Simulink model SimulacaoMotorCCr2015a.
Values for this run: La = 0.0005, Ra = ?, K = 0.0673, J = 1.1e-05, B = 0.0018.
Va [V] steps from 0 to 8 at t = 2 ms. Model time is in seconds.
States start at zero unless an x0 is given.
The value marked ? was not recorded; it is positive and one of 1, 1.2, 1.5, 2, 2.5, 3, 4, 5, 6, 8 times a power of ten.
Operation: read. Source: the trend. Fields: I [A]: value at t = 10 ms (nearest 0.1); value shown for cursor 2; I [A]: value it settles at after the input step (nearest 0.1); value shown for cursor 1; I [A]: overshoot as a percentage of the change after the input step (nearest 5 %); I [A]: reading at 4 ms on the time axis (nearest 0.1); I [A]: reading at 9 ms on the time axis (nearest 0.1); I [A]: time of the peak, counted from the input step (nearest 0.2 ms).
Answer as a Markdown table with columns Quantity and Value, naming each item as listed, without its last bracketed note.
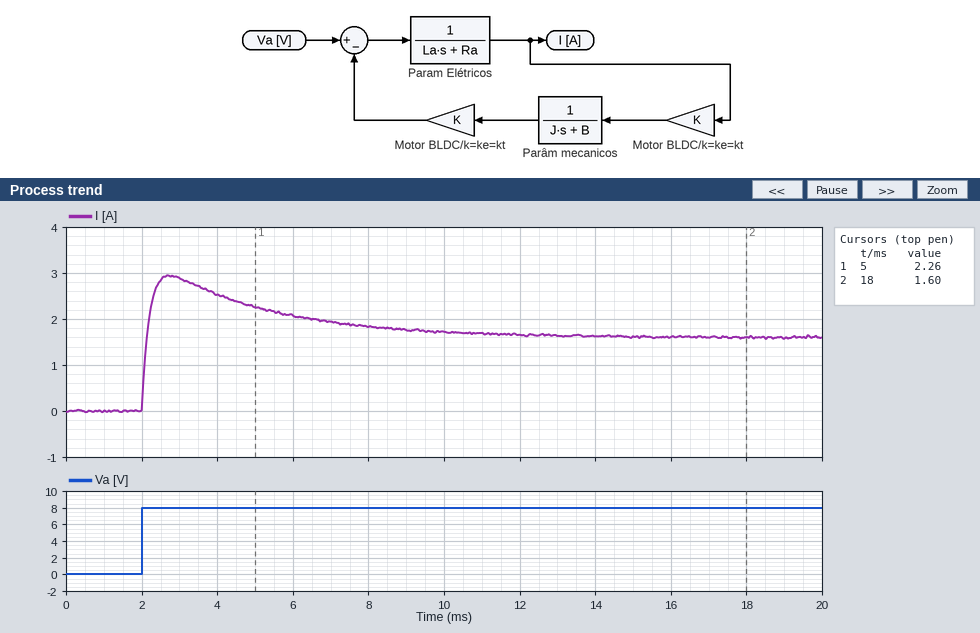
| Quantity | Value |
|---|---|
| I [A]: value at t = 10 ms | 1.7 |
| value shown for cursor 2 | 1.60 |
| I [A]: value it settles at after the input step | 1.6 |
| value shown for cursor 1 | 2.26 |
| I [A]: overshoot as a percentage of the change after the input step | 85 % |
| I [A]: reading at 4 ms on the time axis | 2.5 |
| I [A]: reading at 9 ms on the time axis | 1.8 |
| I [A]: time of the peak, counted from the input step | 0.8 ms |
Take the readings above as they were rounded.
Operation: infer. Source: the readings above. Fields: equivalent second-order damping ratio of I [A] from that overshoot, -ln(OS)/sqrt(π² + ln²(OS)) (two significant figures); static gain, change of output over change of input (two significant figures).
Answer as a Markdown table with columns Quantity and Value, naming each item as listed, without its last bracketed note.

| Quantity | Value |
|---|---|
| equivalent second-order damping ratio of I [A] from that overshoot, -ln(OS)/sqrt(π² + ln²(OS)) | 0.052 |
| static gain, change of output over change of input | 0.20 |
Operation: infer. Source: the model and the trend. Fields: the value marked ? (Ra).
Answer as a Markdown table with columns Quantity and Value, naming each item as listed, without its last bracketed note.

| Quantity | Value |
|---|---|
| the value marked ? | 2.5 |
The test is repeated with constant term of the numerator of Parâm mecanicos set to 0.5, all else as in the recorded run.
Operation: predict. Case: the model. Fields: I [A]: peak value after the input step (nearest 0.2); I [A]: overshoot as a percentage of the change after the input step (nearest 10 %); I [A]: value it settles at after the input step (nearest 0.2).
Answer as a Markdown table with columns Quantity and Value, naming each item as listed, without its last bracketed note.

| Quantity | Value |
|---|---|
| I [A]: peak value after the input step | 3.0 |
| I [A]: overshoot as a percentage of the change after the input step | 40 % |
| I [A]: value it settles at after the input step | 2.2 |
